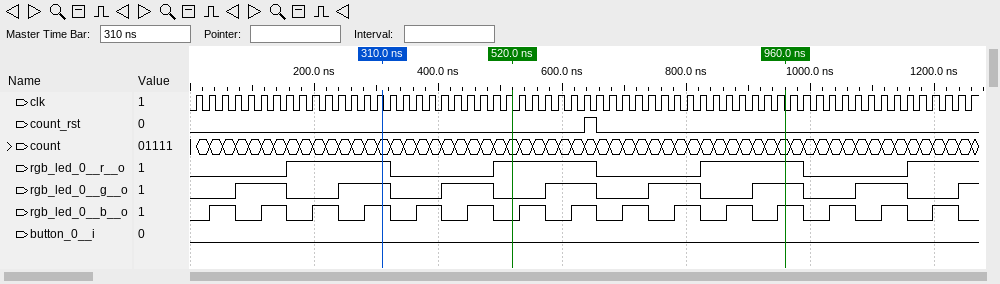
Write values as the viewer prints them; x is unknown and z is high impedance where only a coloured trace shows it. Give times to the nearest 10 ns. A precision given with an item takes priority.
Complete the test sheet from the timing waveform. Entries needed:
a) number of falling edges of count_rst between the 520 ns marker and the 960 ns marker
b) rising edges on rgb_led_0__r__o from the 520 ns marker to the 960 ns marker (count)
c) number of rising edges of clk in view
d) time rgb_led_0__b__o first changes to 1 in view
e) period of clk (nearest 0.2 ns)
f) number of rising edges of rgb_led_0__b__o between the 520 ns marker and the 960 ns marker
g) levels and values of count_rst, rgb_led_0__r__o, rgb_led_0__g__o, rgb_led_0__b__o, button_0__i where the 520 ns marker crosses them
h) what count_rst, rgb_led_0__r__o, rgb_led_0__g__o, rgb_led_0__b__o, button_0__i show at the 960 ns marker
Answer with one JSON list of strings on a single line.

["1", "1", "61", "30 ns", "20.8 ns", "6", "count_rst=0, rgb_led_0__r__o=1, rgb_led_0__g__o=0, rgb_led_0__b__o=0, button_0__i=0", "count_rst=0, rgb_led_0__r__o=1, rgb_led_0__g__o=1, rgb_led_0__b__o=1, button_0__i=0"]
